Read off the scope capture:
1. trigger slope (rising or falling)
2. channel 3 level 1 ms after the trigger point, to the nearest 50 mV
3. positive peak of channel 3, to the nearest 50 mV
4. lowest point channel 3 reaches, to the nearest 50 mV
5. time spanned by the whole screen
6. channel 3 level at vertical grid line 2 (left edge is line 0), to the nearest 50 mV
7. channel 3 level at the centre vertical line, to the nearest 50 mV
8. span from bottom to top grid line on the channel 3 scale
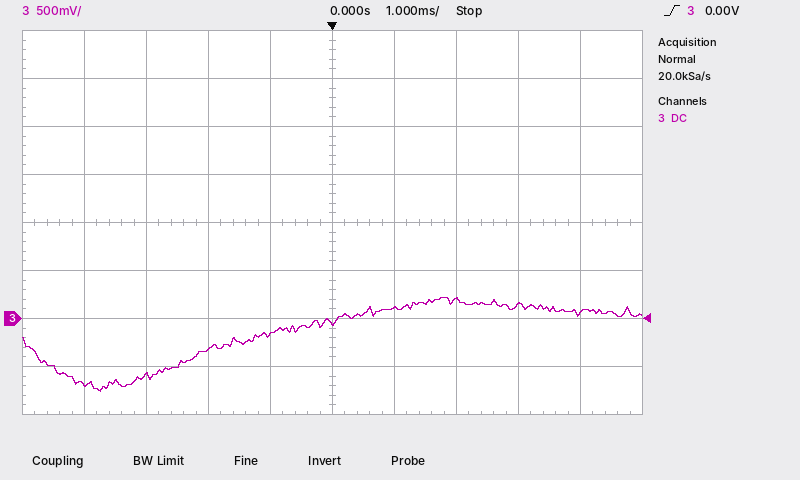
rising
100 mV
200 mV
-750 mV
10 ms
-600 mV
-50 mV
4 V
